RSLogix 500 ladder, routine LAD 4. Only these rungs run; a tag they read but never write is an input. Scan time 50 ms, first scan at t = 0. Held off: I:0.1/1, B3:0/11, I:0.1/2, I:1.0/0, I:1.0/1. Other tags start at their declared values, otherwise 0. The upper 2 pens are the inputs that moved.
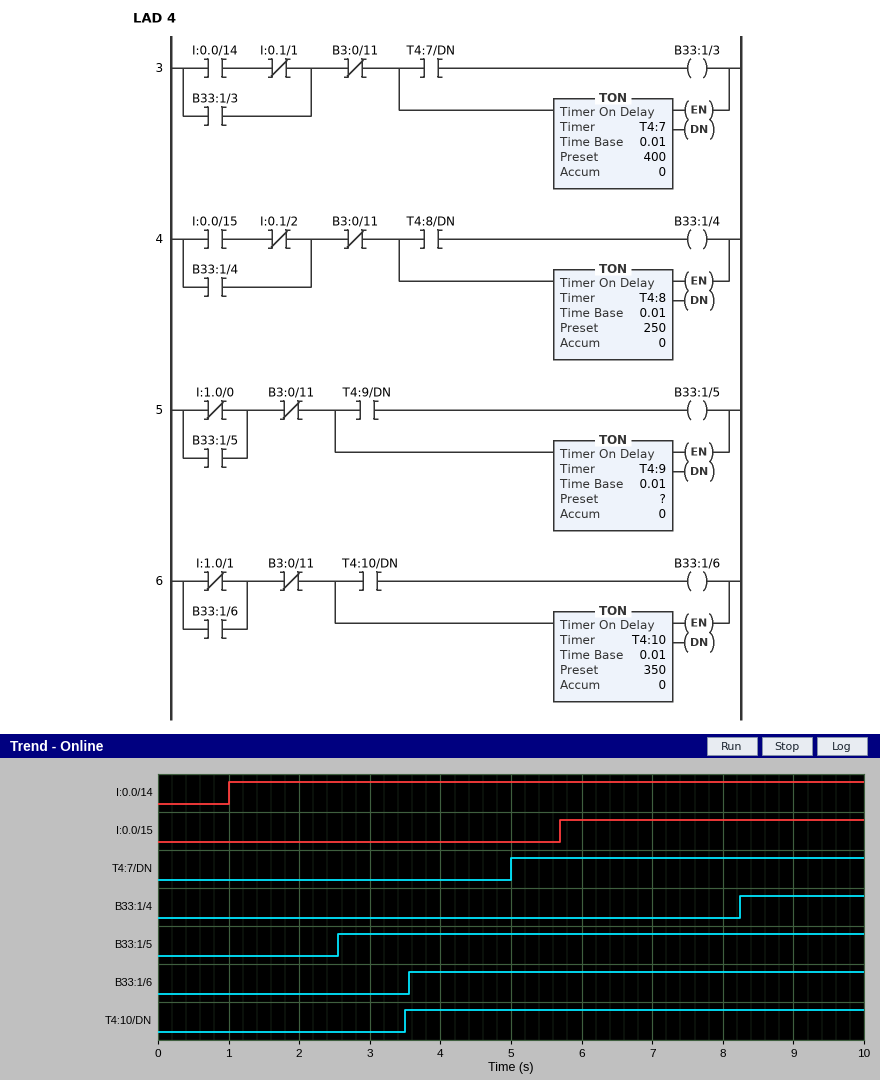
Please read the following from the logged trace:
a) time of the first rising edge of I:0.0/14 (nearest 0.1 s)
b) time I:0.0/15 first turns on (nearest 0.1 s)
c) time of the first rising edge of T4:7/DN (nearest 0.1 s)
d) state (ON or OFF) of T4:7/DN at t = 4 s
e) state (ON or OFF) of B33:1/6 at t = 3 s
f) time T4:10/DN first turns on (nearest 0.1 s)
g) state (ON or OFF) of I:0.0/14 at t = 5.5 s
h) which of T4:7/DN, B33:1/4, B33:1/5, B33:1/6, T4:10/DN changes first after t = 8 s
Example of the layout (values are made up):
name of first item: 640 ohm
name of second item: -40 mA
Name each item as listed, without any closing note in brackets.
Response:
time of the first rising edge of I:0.0/14: 1.0 s
time I:0.0/15 first turns on: 5.7 s
time of the first rising edge of T4:7/DN: 5.0 s
state (ON or OFF) of T4:7/DN at t = 4 s: OFF
state (ON or OFF) of B33:1/6 at t = 3 s: OFF
time T4:10/DN first turns on: 3.5 s
state (ON or OFF) of I:0.0/14 at t = 5.5 s: ON
which of T4:7/DN, B33:1/4, B33:1/5, B33:1/6, T4:10/DN changes first after t = 8 s: B33:1/4
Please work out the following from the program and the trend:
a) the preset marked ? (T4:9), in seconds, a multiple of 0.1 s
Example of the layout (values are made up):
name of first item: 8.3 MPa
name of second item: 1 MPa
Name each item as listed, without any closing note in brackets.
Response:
the preset marked ? (T4:9), in seconds, a multiple of 0.1 s: 2.5 s
